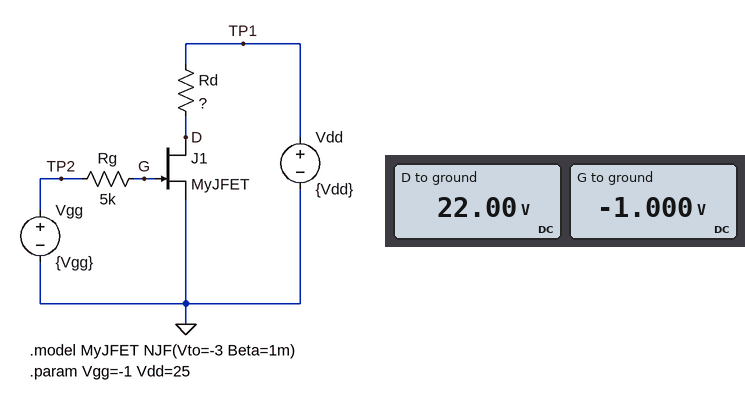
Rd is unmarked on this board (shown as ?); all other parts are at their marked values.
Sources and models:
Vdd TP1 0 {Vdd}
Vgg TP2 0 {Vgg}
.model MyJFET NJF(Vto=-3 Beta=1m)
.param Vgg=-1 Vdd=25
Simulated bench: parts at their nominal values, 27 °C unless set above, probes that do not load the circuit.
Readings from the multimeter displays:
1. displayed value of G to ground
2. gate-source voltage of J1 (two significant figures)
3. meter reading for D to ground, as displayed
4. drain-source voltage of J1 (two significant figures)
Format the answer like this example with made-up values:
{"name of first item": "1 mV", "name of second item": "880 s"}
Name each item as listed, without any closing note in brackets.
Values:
{"displayed value of G to ground": "-1.000 V", "gate-source voltage of J1": "-1.0 V", "meter reading for D to ground, as displayed": "22.00 V", "drain-source voltage of J1": "22 V"}
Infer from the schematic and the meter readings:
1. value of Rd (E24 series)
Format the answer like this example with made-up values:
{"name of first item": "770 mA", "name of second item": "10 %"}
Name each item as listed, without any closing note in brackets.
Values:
{"value of Rd": "750 Ω"}
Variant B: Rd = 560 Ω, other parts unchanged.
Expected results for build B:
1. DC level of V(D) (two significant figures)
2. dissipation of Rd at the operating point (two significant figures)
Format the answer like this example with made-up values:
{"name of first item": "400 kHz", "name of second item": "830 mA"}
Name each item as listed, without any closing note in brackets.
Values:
{"DC level of V(D)": "23 V", "dissipation of Rd at the operating point": "9.0 mW"}
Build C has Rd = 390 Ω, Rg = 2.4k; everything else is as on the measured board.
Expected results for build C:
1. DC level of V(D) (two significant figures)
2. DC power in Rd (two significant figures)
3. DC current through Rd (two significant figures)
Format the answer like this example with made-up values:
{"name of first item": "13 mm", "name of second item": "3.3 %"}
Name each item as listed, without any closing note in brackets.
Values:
{"DC level of V(D)": "23 V", "DC power in Rd": "6.2 mW", "DC current through Rd": "4.0 mA"}
